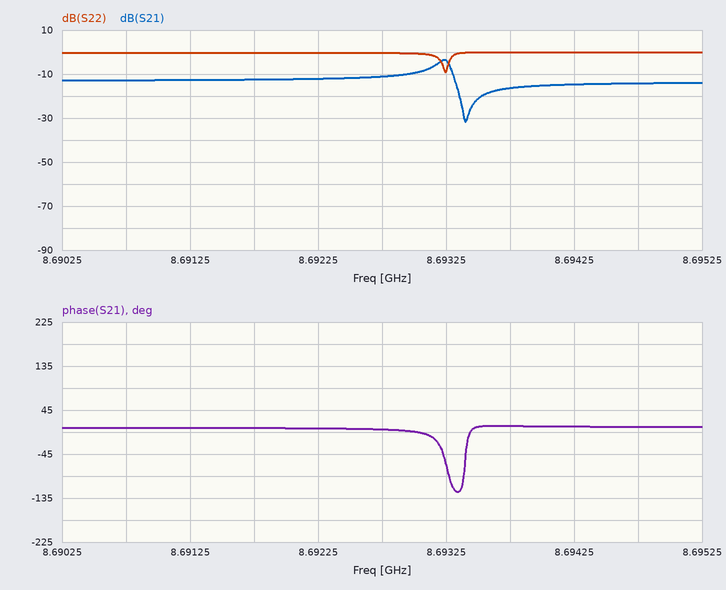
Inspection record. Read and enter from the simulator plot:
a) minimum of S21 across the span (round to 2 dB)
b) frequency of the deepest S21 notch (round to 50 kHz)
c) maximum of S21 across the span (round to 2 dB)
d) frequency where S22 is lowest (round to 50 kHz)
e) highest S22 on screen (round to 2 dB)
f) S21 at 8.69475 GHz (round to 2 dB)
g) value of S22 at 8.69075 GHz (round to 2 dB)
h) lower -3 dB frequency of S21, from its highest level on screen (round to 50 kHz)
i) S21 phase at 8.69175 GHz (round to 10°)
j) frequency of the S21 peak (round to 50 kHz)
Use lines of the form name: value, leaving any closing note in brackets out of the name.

minimum of S21 across the span: -32 dB
frequency of the deepest S21 notch: 8.69340 GHz
maximum of S21 across the span: -4 dB
frequency where S22 is lowest: 8.69325 GHz
highest S22 on screen: 0 dB
S21 at 8.69475 GHz: -14 dB
value of S22 at 8.69075 GHz: 0 dB
lower -3 dB frequency of S21, from its highest level on screen: 8.69315 GHz
S21 phase at 8.69175 GHz: 10°
frequency of the S21 peak: 8.69325 GHz
